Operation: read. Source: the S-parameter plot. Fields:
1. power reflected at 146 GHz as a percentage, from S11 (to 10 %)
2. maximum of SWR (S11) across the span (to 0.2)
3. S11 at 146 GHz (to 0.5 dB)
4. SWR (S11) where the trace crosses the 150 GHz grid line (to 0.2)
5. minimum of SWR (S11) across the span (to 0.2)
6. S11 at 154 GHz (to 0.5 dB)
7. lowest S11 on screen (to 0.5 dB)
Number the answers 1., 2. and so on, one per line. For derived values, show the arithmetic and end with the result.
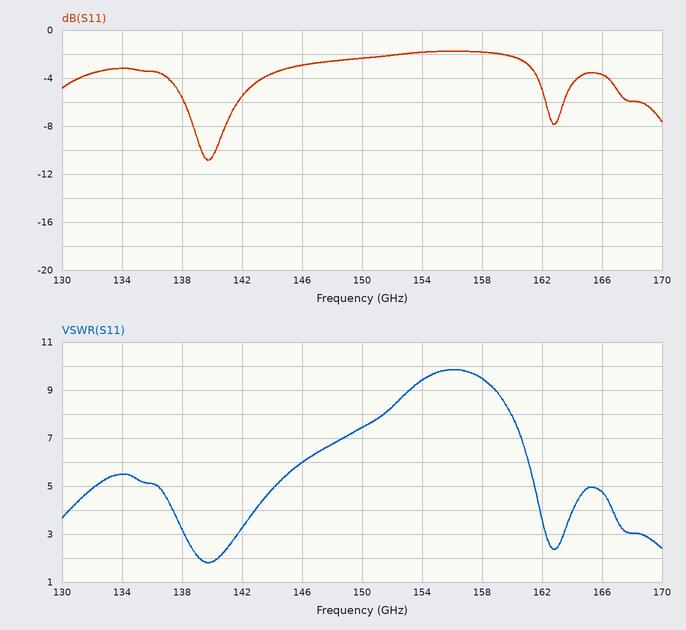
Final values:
1. 10^(-3/10) ≈ 50 %
2. 9.8
3. -3.0 dB
4. 7.4
5. 1.8
6. -2.0 dB
7. -11.0 dB
